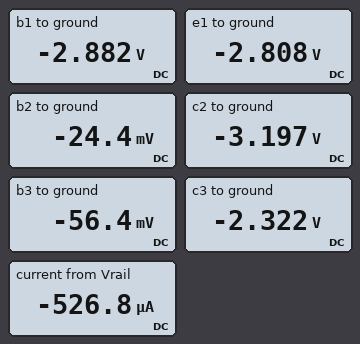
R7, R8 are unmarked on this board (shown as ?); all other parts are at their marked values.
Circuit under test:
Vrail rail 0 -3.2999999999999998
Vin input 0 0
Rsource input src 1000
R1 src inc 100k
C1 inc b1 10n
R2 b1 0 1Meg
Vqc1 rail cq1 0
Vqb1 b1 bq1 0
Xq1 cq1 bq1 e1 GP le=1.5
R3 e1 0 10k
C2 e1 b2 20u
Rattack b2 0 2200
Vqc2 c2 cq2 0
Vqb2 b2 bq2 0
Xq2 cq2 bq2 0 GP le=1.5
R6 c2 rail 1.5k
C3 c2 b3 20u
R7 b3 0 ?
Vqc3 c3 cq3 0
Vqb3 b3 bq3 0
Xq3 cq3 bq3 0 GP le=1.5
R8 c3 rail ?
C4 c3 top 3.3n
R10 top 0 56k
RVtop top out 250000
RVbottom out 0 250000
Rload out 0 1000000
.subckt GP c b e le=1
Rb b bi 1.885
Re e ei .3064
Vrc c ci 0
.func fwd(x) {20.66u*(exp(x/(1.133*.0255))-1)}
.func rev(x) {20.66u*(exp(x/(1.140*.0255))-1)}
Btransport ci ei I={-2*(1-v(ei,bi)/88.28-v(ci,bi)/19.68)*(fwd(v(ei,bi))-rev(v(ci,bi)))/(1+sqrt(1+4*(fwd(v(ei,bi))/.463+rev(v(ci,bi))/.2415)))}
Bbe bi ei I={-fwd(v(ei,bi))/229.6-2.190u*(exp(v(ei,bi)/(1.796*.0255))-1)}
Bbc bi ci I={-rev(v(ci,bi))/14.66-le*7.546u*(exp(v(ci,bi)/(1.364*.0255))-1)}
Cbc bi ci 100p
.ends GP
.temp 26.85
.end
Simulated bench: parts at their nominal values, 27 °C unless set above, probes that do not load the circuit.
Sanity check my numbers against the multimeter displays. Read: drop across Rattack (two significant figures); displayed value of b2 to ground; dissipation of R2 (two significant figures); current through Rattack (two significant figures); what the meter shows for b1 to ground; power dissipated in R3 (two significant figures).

24 mV
-24.4 mV
8.3 µW
11 µA
-2.882 V
790 µW
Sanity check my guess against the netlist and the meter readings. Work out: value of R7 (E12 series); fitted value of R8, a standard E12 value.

8.2 kΩ
5.6 kΩ
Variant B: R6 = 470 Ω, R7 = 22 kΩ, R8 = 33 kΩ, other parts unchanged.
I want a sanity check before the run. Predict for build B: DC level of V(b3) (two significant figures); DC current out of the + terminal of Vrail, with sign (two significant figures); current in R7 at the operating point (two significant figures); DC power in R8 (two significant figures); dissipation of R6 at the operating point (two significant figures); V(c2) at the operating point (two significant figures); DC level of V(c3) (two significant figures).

-46 mV
-450 µA
2.1 µA
320 µW
2.2 µW
-3.3 V
-69 mV
